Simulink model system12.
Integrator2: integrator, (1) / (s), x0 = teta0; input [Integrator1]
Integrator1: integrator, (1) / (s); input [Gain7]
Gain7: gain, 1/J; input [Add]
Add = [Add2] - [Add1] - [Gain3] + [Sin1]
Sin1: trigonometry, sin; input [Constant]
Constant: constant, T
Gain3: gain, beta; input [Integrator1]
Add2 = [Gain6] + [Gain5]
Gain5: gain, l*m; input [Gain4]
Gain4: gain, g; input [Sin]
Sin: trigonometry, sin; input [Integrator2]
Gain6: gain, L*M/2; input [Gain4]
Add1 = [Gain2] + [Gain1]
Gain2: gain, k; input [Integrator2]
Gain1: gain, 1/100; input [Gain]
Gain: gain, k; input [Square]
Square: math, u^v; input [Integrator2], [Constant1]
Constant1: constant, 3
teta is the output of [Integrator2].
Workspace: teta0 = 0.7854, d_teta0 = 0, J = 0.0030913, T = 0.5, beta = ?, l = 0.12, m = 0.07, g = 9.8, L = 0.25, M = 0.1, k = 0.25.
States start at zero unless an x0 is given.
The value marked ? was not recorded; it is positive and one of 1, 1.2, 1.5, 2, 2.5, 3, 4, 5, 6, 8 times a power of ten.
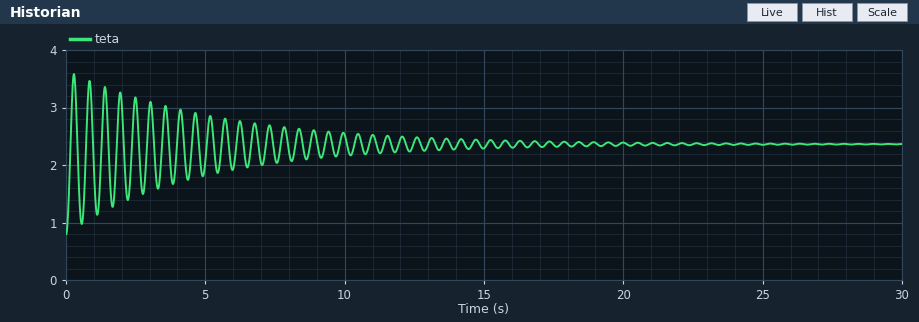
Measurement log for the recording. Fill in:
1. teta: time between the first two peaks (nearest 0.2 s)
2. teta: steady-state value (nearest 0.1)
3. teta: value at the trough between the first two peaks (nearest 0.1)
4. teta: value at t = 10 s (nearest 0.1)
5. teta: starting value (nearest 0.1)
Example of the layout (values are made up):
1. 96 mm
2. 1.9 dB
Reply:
1. 0.6 s
2. 2.4
3. 1.0
4. 2.5
5. 0.8
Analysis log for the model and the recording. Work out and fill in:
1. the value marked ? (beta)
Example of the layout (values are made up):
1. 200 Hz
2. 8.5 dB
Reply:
1. 0.0012
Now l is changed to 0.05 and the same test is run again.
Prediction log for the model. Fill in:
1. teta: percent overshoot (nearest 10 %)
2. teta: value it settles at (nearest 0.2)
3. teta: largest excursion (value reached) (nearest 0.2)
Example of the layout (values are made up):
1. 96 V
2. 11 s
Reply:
1. 80 %
2. 2.2
3. 3.4
